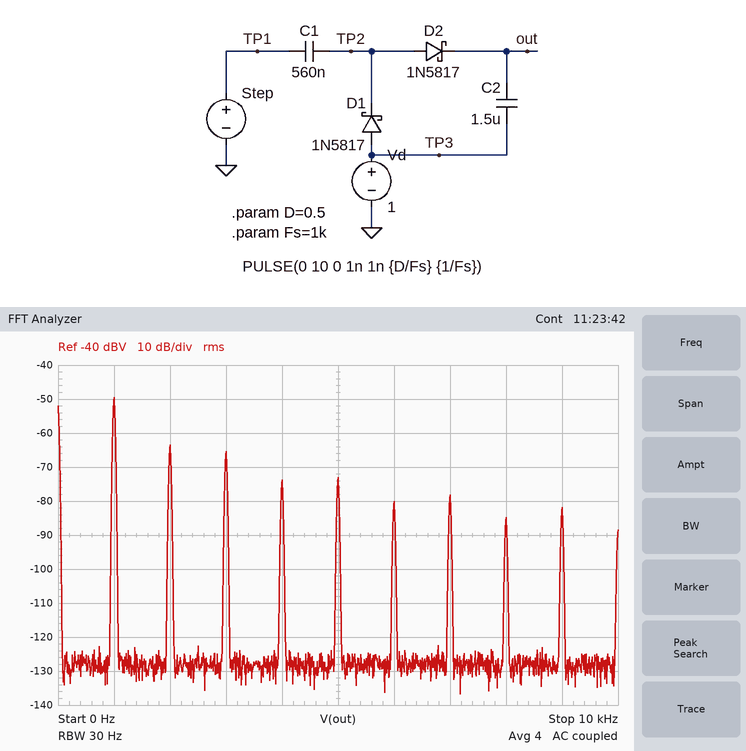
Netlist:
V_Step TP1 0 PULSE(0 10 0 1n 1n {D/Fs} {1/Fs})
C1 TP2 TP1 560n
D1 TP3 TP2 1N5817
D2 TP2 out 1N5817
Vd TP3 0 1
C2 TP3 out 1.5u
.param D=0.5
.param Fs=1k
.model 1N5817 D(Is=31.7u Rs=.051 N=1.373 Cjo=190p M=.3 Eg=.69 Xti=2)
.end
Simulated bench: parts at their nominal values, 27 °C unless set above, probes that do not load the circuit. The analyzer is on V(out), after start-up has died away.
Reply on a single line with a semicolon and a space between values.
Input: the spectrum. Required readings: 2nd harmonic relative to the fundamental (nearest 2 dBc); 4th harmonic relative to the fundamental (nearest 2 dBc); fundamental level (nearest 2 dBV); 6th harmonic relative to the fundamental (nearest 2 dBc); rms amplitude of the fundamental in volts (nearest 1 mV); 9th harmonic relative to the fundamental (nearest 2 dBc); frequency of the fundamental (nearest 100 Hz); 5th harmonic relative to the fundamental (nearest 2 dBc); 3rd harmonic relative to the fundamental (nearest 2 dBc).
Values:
-14 dBc; -24 dBc; -50 dBV; -30 dBc; 3 mV; -32 dBc; 1.0 kHz; -24 dBc; -16 dBc
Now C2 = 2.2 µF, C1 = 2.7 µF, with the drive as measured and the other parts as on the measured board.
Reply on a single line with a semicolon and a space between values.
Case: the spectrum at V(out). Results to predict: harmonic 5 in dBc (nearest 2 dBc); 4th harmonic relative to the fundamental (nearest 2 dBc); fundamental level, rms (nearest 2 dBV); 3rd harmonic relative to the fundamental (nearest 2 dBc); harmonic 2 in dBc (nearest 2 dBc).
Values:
-26 dBc; -36 dBc; -54 dBV; -18 dBc; -24 dBc
